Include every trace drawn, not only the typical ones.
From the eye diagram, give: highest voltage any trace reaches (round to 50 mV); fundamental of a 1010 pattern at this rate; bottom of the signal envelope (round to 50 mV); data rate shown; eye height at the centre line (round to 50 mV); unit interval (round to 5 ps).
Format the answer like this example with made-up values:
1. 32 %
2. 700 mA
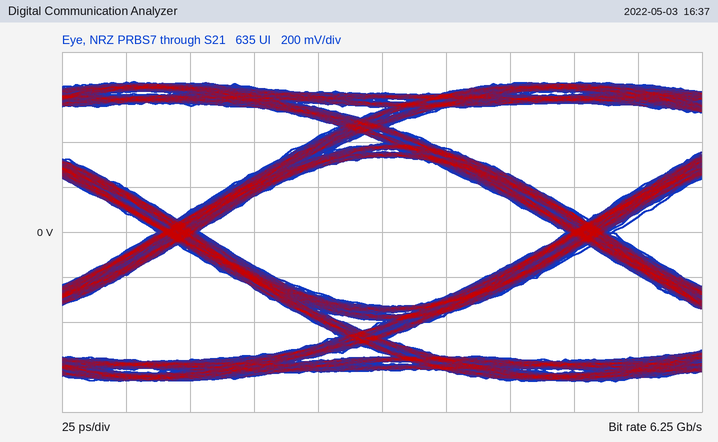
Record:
1. 650 mV
2. 3.125 GHz
3. -650 mV
4. 6.25 Gb/s
5. 650 mV
6. 160 ps
